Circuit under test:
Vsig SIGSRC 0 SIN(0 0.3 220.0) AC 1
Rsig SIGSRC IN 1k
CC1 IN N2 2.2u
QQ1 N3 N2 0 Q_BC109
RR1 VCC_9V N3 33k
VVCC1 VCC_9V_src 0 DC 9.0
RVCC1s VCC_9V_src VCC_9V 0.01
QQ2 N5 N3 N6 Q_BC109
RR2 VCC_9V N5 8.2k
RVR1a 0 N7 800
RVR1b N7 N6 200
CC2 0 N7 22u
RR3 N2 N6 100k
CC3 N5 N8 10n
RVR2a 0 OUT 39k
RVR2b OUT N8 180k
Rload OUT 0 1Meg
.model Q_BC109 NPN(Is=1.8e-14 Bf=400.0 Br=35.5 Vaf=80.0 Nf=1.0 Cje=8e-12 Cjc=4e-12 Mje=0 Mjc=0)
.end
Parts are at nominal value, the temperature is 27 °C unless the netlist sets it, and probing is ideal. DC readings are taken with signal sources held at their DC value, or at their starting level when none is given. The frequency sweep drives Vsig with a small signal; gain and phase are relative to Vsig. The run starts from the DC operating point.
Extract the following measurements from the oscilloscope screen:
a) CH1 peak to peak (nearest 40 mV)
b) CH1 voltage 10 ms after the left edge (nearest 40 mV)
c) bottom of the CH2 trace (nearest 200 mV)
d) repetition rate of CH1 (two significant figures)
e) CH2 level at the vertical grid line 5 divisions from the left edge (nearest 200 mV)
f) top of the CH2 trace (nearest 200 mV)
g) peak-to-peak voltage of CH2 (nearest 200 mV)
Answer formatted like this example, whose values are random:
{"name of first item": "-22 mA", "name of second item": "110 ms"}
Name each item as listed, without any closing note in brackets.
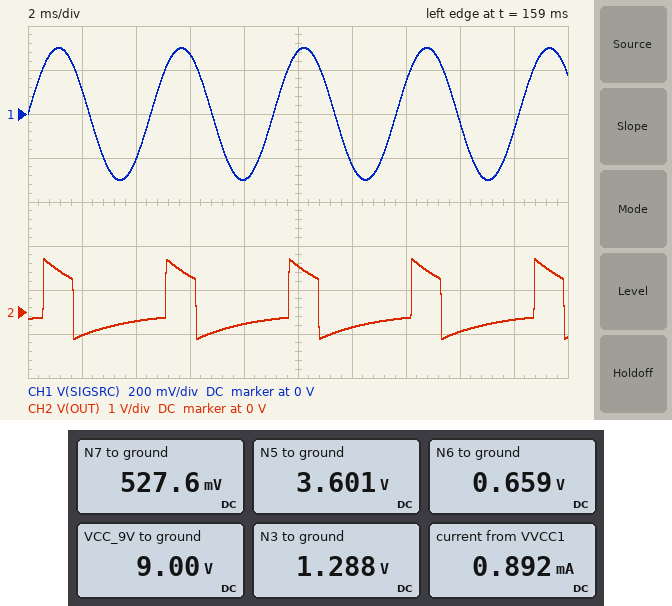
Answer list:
{"CH1 peak to peak": "600 mV", "CH1 voltage 10 ms after the left edge": "280 mV", "bottom of the CH2 trace": "-600 mV", "repetition rate of CH1": "220 Hz", "CH2 level at the vertical grid line 5 divisions from the left edge": "1.0 V", "top of the CH2 trace": "1.2 V", "peak-to-peak voltage of CH2": "1.8 V"}
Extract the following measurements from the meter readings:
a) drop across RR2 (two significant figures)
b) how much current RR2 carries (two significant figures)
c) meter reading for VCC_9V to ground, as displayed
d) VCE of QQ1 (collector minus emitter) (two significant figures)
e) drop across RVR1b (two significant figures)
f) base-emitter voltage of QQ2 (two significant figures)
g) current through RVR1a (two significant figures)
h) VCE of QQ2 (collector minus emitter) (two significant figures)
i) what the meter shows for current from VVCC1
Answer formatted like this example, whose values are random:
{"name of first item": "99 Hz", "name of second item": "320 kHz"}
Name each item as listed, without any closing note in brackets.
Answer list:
{"drop across RR2": "5.4 V", "how much current RR2 carries": "660 µA", "meter reading for VCC_9V to ground, as displayed": "9.00 V", "VCE of QQ1 (collector minus emitter)": "1.3 V", "drop across RVR1b": "130 mV", "base-emitter voltage of QQ2": "630 mV", "current through RVR1a": "660 µA", "VCE of QQ2 (collector minus emitter)": "2.9 V", "what the meter shows for current from VVCC1": "0.892 mA"}
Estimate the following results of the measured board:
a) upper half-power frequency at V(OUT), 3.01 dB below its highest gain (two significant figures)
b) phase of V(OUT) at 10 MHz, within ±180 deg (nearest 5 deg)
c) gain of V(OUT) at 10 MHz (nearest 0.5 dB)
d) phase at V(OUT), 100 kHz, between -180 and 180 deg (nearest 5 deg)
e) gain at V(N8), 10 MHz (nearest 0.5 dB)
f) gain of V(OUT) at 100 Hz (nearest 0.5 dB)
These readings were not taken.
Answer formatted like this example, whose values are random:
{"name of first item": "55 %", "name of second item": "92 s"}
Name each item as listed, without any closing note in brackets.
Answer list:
{"upper half-power frequency at V(OUT), 3.01 dB below its highest gain": "100 kHz", "phase of V(OUT) at 10 MHz, within ±180 deg": "-140 deg", "gain of V(OUT) at 10 MHz": "10.0 dB", "phase at V(OUT), 100 kHz, between -180 and 180 deg": "-45 deg", "gain at V(N8), 10 MHz": "25.0 dB", "gain of V(OUT) at 100 Hz": "49.5 dB"}
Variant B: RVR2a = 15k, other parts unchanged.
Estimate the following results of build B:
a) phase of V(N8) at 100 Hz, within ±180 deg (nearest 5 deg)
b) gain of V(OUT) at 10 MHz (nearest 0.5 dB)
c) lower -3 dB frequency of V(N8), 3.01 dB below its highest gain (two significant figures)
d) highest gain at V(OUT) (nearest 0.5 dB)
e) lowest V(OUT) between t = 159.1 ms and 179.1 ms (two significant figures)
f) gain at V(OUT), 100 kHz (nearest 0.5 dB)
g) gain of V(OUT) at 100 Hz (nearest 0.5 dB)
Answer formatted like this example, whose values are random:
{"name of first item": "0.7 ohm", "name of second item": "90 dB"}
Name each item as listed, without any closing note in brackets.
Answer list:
{"phase of V(N8) at 100 Hz, within ±180 deg": "80 deg", "gain of V(OUT) at 10 MHz": "3.0 dB", "lower -3 dB frequency of V(N8), 3.01 dB below its highest gain": "110 Hz", "highest gain at V(OUT)": "45.5 dB", "lowest V(OUT) between t = 159.1 ms and 179.1 ms": "-290 mV", "gain at V(OUT), 100 kHz": "42.5 dB", "gain of V(OUT) at 100 Hz": "42.0 dB"}
